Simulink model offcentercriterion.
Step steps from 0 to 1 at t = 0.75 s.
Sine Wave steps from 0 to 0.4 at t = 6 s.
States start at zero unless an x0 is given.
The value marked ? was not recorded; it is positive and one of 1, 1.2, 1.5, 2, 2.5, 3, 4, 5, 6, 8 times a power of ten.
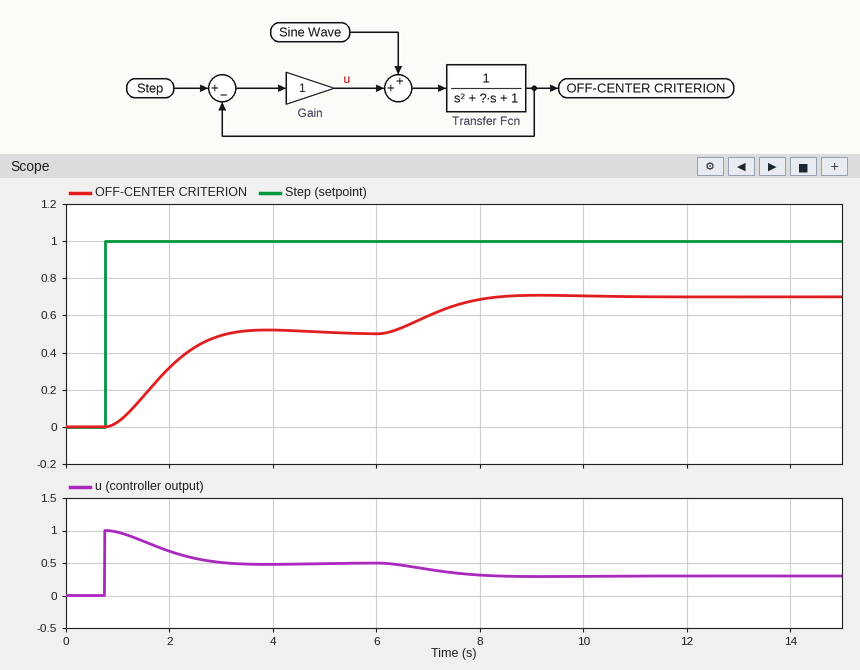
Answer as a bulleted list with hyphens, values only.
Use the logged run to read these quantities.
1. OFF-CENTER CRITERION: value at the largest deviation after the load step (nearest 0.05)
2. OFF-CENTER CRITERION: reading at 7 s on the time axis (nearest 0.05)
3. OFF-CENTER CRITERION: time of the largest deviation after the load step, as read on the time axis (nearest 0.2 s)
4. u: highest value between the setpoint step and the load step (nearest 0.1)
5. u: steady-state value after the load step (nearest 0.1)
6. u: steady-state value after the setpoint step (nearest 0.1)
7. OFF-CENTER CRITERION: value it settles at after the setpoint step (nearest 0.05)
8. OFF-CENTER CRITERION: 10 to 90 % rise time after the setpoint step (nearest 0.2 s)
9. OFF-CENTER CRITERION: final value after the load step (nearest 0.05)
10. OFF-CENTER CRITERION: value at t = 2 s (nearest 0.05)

- 0.70
- 0.60
- 9.2 s
- 1.0
- 0.3
- 0.5
- 0.50
- 1.6 s
- 0.70
- 0.30
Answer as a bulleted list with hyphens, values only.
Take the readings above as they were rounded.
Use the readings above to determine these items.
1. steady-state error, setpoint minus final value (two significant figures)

- 0.50
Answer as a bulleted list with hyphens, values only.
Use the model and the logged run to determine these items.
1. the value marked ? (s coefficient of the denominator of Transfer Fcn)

- 2
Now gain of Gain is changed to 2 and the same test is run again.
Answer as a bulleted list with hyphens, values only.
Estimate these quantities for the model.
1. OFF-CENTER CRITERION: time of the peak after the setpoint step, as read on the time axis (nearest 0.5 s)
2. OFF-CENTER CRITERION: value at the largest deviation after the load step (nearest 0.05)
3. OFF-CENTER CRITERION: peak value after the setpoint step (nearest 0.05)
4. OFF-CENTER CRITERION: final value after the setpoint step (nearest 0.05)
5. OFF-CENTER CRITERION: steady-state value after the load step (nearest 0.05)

- 3.0 s
- 0.80
- 0.75
- 0.65
- 0.80
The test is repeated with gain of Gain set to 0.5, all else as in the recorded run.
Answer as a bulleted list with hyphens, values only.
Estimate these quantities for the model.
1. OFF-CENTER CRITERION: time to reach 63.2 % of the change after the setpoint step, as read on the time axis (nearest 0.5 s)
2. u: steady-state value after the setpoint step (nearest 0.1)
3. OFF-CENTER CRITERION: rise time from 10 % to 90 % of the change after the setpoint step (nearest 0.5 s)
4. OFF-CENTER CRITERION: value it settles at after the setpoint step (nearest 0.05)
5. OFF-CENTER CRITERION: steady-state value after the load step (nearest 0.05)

- 2.5 s
- 0.3
- 2.0 s
- 0.35
- 0.60
